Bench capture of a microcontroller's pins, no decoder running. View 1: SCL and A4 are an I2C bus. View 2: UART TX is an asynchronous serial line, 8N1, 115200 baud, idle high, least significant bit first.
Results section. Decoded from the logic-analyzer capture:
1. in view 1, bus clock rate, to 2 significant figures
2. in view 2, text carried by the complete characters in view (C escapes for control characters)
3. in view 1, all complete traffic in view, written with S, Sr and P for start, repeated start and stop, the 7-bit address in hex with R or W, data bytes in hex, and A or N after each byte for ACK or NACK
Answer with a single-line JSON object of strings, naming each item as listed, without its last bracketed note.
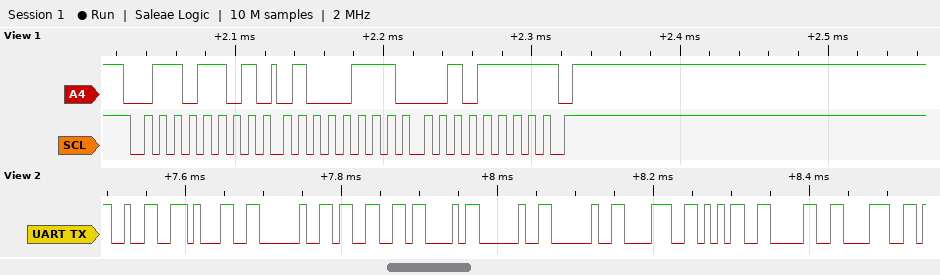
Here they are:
{"in view 1, bus clock rate, to 2 significant figures": "100 kHz", "in view 2, text carried by the complete characters in view": "\"21 3C  8508\"", "in view 1, all complete traffic in view, written with S, Sr and P for start, repeated start and stop, the 7-bit address in hex with R or W, data bytes in hex, and A or N after each byte for ACK or NACK": "S 36R A 47 A 2F N P"}
